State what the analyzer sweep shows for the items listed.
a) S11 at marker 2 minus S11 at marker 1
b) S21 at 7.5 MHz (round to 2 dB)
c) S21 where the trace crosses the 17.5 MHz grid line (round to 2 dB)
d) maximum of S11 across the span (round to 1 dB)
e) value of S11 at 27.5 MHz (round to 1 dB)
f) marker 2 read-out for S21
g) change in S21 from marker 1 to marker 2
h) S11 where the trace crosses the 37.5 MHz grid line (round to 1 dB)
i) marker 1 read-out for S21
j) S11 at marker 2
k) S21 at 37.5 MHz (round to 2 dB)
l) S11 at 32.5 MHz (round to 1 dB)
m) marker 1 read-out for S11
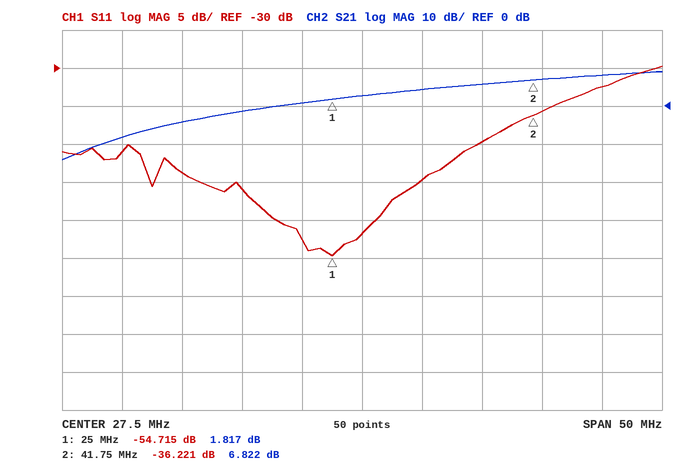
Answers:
18.494 dB
-8 dB
-2 dB
-30 dB
-52 dB
6.822 dB
5.005 dB
-40 dB
1.817 dB
-36.221 dB
6 dB
-45 dB
-54.715 dB
